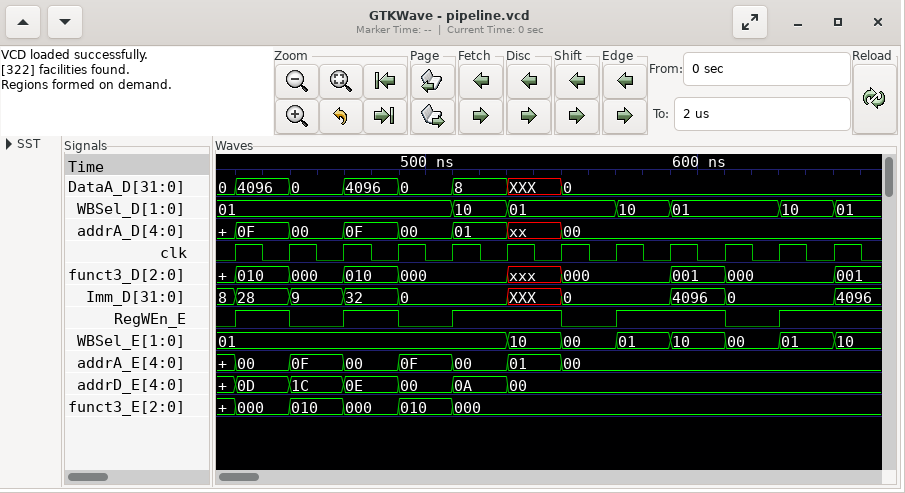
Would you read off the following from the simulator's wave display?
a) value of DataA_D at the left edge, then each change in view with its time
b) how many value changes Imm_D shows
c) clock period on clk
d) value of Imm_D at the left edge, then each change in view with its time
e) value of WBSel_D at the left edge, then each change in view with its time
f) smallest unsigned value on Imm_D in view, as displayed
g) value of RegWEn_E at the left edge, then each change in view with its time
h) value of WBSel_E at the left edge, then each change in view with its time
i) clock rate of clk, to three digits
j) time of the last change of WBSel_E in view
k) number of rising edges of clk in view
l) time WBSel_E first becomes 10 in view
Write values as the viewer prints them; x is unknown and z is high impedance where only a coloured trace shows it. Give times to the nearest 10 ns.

0, 4096 at 430 ns, 0 at 450 ns, 4096 at 470 ns, 0 at 490 ns, 8 at 510 ns, XXX at 530 ns, 0 at 550 ns
9
20 ns
8, 28 at 430 ns, 9 at 450 ns, 32 at 470 ns, 0 at 490 ns, XXX at 530 ns, 0 at 550 ns, 4096 at 590 ns, 0 at 610 ns, 4096 at 650 ns
01, 10 at 510 ns, 01 at 530 ns, 10 at 570 ns, 01 at 590 ns, 10 at 630 ns, 01 at 650 ns
0
0, 1 at 430 ns, 0 at 450 ns, 1 at 470 ns, 0 at 490 ns, 1 at 510 ns, 0 at 550 ns, 1 at 570 ns, 0 at 610 ns, 1 at 630 ns
01, 10 at 530 ns, 00 at 550 ns, 01 at 570 ns, 10 at 590 ns, 00 at 610 ns, 01 at 630 ns, 10 at 650 ns
50.0 MHz
650 ns
12
530 ns
